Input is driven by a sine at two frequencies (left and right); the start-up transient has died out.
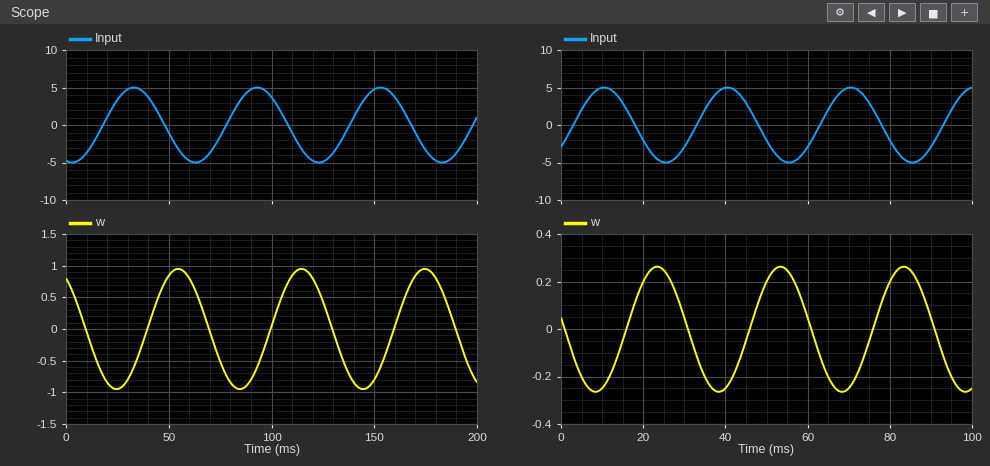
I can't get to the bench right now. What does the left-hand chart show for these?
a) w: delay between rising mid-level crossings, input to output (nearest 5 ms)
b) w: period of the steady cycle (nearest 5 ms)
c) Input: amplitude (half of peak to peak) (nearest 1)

20 ms
60 ms
5
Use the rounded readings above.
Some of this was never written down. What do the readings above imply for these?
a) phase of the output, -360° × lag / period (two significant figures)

-120°
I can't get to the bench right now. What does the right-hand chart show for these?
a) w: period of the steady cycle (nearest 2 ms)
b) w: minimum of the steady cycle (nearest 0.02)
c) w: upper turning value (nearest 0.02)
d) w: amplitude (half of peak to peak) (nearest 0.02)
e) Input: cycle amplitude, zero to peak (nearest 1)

30 ms
-0.26
0.26
0.26
5
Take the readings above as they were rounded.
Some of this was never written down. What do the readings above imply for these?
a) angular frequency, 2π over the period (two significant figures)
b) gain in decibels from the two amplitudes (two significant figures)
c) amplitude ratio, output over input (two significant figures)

0.21 rad/ms
-26 dB
0.052
